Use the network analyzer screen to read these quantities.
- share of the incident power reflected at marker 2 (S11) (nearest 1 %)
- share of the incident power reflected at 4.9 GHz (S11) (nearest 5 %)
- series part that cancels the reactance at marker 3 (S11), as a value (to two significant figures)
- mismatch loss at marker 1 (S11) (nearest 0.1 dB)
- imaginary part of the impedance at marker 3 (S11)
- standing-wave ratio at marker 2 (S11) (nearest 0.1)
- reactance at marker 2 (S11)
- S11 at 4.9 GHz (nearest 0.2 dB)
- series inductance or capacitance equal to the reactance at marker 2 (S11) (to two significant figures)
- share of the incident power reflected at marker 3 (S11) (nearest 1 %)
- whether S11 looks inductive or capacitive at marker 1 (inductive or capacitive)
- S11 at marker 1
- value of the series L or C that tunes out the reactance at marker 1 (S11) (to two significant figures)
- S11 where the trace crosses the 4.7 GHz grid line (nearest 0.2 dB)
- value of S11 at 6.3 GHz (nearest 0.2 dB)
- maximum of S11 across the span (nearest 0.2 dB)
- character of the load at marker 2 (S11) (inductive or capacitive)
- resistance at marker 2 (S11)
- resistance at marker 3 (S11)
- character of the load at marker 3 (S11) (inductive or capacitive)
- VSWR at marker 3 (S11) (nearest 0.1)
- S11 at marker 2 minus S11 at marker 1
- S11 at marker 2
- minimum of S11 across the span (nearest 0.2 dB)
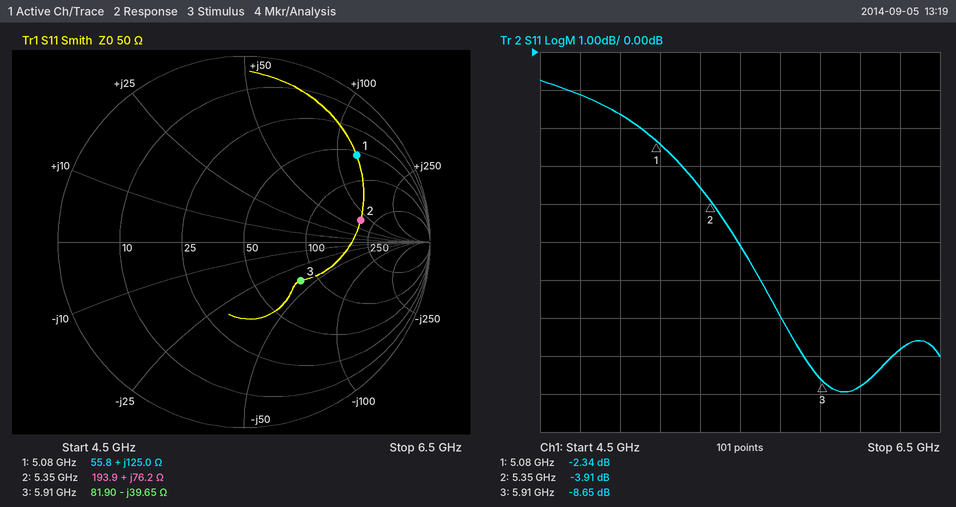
41 %
70 %
1.1 nH
3.8 dB
-39.65 Ω
4.5
+76.2 Ω
-1.6 dB
2.3 nH
14 %
inductive
-2.34 dB
250 fF
-1.2 dB
-7.8 dB
-0.8 dB
inductive
193.9 Ω
81.90 Ω
capacitive
2.2
-1.57 dB
-3.91 dB
-9.0 dB
